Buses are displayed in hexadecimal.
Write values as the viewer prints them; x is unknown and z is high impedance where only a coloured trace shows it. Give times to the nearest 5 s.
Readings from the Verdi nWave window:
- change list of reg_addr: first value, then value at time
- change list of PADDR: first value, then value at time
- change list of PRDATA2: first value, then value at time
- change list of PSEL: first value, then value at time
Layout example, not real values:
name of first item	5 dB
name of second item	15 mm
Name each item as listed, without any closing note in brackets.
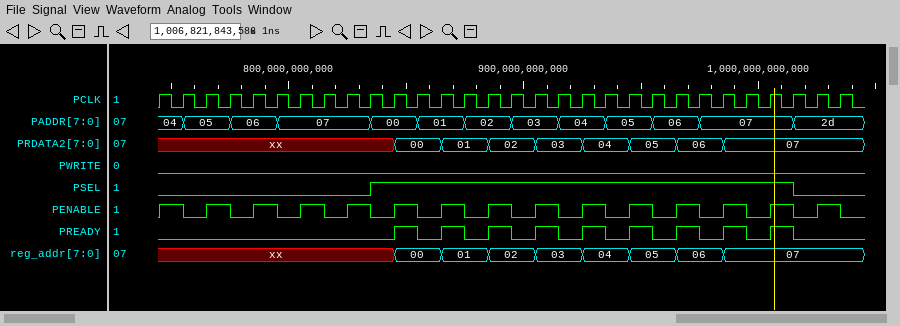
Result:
change list of reg_addr: first value, then value at time	xx, 00 at 845 s, 01 at 865 s, 02 at 885 s, 03 at 905 s, 04 at 925 s, 05 at 945 s, 06 at 965 s, 07 at 985 s
change list of PADDR: first value, then value at time	04, 05 at 755 s, 06 at 775 s, 07 at 795 s, 00 at 835 s, 01 at 855 s, 02 at 875 s, 03 at 895 s, 04 at 915 s, 05 at 935 s, 06 at 955 s, 07 at 975 s, 2d at 1015 s
change list of PRDATA2: first value, then value at time	xx, 00 at 845 s, 01 at 865 s, 02 at 885 s, 03 at 905 s, 04 at 925 s, 05 at 945 s, 06 at 965 s, 07 at 985 s
change list of PSEL: first value, then value at time	0, 1 at 835 s, 0 at 1015 s
